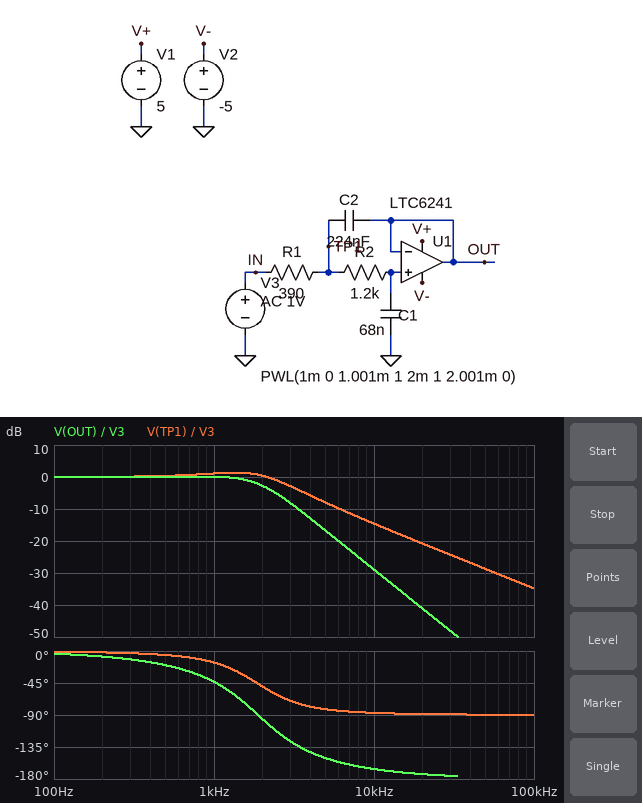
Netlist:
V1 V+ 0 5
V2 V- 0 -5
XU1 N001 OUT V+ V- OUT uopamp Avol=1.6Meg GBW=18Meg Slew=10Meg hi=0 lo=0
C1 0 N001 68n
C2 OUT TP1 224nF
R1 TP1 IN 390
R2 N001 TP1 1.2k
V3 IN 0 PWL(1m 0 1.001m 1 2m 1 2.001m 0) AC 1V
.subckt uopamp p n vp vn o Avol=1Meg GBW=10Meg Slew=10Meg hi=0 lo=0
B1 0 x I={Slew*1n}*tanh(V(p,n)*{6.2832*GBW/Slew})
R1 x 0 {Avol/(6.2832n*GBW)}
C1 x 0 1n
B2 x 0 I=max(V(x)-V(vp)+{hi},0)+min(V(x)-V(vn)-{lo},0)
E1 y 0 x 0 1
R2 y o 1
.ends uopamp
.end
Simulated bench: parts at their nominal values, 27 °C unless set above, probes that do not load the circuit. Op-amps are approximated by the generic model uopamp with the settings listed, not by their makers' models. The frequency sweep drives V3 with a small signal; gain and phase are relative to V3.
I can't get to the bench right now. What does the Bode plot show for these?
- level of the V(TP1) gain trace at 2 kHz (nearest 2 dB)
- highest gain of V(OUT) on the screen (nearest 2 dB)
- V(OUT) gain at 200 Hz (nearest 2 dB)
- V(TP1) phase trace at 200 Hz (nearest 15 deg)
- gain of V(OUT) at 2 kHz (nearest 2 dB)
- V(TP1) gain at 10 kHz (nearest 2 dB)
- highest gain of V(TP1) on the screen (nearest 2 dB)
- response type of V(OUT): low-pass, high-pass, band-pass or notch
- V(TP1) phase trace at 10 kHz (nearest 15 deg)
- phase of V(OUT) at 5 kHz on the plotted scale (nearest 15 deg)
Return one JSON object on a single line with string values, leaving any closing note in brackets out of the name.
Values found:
{"level of the V(TP1) gain trace at 2 kHz": "0 dB", "highest gain of V(OUT) on the screen": "0 dB", "V(OUT) gain at 200 Hz": "0 dB", "V(TP1) phase trace at 200 Hz": "0 deg", "gain of V(OUT) at 2 kHz": "-2 dB", "V(TP1) gain at 10 kHz": "-14 dB", "highest gain of V(TP1) on the screen": "2 dB", "response type of V(OUT): low-pass, high-pass, band-pass or notch": "low-pass", "V(TP1) phase trace at 10 kHz": "-90 deg", "phase of V(OUT) at 5 kHz on the plotted scale": "-150 deg"}
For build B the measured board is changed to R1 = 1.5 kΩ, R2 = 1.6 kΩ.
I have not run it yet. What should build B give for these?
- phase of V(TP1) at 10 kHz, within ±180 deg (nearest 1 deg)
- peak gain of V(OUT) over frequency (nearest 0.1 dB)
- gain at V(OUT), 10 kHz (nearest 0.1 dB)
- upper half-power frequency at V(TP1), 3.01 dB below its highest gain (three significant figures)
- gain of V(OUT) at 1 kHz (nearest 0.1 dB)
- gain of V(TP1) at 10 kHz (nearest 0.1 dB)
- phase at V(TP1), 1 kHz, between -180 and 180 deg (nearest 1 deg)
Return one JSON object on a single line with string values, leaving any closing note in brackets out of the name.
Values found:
{"phase of V(TP1) at 10 kHz, within ±180 deg": "-93 deg", "peak gain of V(OUT) over frequency": "0.7 dB", "gain at V(OUT), 10 kHz": "-43.2 dB", "upper half-power frequency at V(TP1), 3.01 dB below its highest gain": "1.04 kHz", "gain of V(OUT) at 1 kHz": "-2.9 dB", "gain of V(TP1) at 10 kHz": "-26.4 dB", "phase at V(TP1), 1 kHz, between -180 and 180 deg": "-74 deg"}
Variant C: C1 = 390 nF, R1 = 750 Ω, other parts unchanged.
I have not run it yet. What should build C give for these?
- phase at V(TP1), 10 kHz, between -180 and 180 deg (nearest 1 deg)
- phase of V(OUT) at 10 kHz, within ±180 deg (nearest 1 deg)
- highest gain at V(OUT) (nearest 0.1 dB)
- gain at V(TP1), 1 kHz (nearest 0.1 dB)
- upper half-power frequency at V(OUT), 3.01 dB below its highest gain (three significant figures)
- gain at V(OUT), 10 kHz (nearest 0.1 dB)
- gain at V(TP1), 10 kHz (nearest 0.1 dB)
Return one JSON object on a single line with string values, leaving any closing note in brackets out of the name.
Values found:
{"phase at V(TP1), 10 kHz, between -180 and 180 deg": "-83 deg", "phase of V(OUT) at 10 kHz, within ±180 deg": "-171 deg", "highest gain at V(OUT)": "0 dB", "gain at V(TP1), 1 kHz": "-4.5 dB", "upper half-power frequency at V(OUT), 3.01 dB below its highest gain": "241 Hz", "gain at V(OUT), 10 kHz": "-49.9 dB", "gain at V(TP1), 10 kHz": "-20.5 dB"}
